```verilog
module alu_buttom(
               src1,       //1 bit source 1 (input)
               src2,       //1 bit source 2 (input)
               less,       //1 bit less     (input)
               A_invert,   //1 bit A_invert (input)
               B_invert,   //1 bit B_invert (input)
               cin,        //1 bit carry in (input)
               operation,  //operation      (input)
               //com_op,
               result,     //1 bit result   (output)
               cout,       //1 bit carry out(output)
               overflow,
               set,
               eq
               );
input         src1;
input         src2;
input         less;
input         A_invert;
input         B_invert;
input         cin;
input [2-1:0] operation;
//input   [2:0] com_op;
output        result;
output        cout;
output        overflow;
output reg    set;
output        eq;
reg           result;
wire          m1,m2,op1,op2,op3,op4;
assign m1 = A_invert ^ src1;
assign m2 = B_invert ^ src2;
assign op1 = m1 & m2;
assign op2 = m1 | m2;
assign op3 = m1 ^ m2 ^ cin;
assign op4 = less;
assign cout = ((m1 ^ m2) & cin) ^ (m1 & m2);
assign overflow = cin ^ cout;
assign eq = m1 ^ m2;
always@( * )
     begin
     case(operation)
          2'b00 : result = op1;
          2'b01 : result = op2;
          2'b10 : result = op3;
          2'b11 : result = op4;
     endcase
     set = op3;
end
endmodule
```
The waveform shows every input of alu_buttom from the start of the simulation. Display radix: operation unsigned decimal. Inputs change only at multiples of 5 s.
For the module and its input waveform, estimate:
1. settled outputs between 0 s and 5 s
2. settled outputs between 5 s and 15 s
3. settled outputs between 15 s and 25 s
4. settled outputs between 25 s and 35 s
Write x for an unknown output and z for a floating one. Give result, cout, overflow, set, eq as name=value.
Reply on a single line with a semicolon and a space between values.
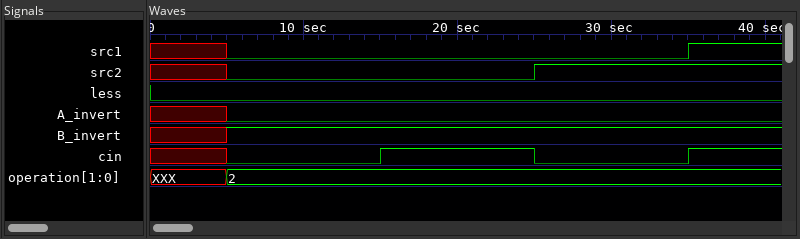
result=x, cout=x, overflow=x, set=x, eq=x; result=1, cout=0, overflow=0, set=1, eq=1; result=0, cout=1, overflow=0, set=0, eq=1; result=0, cout=0, overflow=0, set=0, eq=0
